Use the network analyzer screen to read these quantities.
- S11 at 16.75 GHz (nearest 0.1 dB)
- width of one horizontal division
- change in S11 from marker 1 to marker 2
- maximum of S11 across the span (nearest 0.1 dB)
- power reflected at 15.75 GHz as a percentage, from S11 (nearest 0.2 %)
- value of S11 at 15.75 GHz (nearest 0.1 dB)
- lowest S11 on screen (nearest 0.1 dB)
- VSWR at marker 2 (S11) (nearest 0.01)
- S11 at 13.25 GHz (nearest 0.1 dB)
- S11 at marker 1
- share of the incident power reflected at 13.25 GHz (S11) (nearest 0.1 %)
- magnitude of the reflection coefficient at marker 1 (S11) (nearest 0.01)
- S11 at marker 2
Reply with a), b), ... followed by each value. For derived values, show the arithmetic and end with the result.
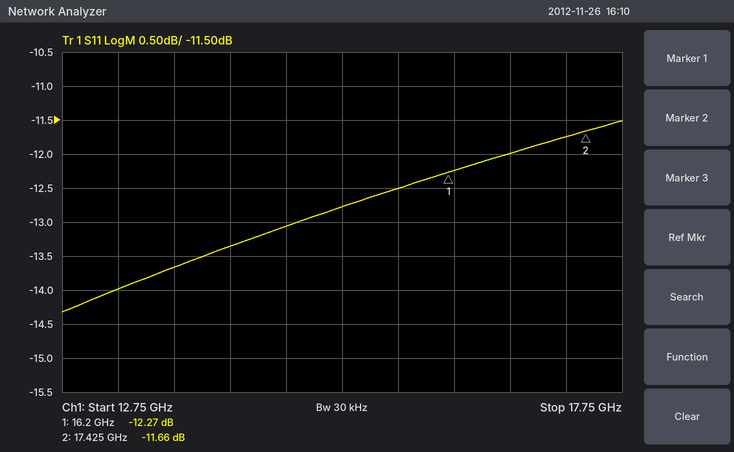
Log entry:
a) -12.0 dB
b) 500 MHz
c) -11.66 − (-12.27) = 0.61 dB
d) -11.5 dB
e) 10^(-12.5/10) ≈ 5.6 %
f) -12.5 dB
g) -14.3 dB
h) (1 + 0.2612)/(1 − 0.2612) ≈ 1.71
i) -14.0 dB
j) -12.27 dB
k) 10^(-14/10) ≈ 4.0 %
l) 10^(-12.27/20) ≈ 0.24
m) -11.66 dB
